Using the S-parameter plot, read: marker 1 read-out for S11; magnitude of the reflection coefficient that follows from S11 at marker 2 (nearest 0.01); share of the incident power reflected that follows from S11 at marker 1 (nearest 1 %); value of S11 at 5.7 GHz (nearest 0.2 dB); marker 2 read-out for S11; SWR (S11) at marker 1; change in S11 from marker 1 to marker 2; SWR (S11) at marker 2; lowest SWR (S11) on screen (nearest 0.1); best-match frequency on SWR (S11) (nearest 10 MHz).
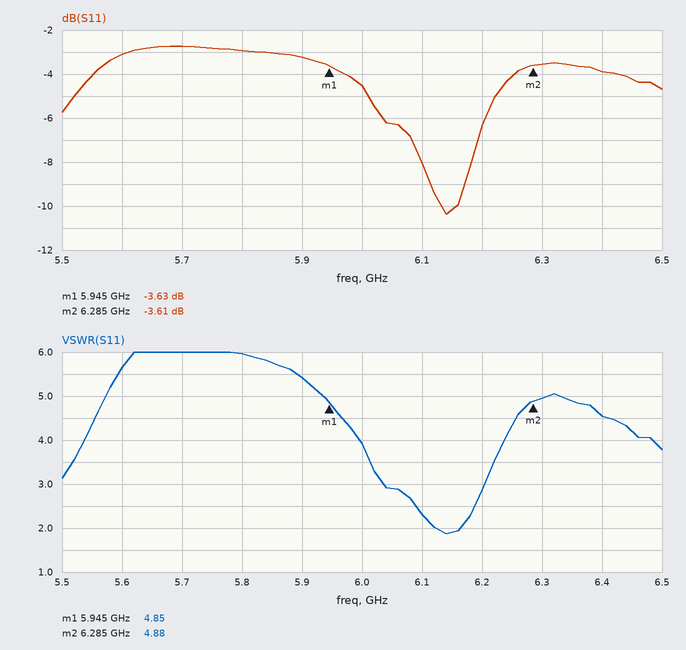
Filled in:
-3.63 dB
0.66
43 %
-2.8 dB
-3.61 dB
4.85
0.02 dB
4.88
1.9
6.14 GHz
